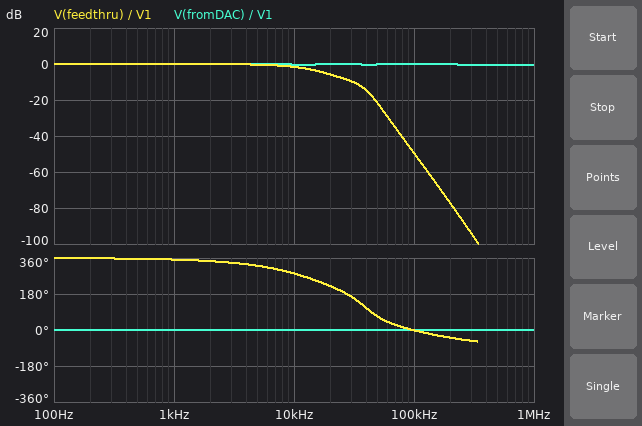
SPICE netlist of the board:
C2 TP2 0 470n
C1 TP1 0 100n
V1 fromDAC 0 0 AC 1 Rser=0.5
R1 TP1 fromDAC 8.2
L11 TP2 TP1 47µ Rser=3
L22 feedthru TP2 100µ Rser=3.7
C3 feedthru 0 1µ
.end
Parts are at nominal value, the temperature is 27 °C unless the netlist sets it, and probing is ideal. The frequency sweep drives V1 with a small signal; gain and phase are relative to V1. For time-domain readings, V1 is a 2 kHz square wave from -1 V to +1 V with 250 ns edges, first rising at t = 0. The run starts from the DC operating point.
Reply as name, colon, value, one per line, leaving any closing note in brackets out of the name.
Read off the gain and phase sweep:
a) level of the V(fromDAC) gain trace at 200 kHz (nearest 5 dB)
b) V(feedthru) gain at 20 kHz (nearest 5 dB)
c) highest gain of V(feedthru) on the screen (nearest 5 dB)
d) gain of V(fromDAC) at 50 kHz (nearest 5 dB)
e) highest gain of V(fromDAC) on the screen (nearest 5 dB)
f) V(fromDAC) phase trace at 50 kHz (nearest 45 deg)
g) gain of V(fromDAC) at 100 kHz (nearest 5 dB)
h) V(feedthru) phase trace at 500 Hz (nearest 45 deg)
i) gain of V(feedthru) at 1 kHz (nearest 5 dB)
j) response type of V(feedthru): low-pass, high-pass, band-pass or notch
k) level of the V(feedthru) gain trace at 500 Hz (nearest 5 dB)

level of the V(fromDAC) gain trace at 200 kHz: 0 dB
V(feedthru) gain at 20 kHz: -5 dB
highest gain of V(feedthru) on the screen: 0 dB
gain of V(fromDAC) at 50 kHz: 0 dB
highest gain of V(fromDAC) on the screen: 0 dB
V(fromDAC) phase trace at 50 kHz: 0 deg
gain of V(fromDAC) at 100 kHz: 0 dB
V(feedthru) phase trace at 500 Hz: 360 deg
gain of V(feedthru) at 1 kHz: 0 dB
response type of V(feedthru): low-pass, high-pass, band-pass or notch: low-pass
level of the V(feedthru) gain trace at 500 Hz: 0 dB
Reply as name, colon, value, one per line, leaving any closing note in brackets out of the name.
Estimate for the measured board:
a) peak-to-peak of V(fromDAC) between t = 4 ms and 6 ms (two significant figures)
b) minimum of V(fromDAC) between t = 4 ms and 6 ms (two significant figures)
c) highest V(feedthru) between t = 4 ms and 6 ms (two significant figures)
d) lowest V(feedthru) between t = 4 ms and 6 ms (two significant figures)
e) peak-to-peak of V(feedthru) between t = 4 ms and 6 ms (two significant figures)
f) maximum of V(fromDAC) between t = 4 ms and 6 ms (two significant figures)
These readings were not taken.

peak-to-peak of V(fromDAC) between t = 4 ms and 6 ms: 2.0 V
minimum of V(fromDAC) between t = 4 ms and 6 ms: -1.0 V
highest V(feedthru) between t = 4 ms and 6 ms: 1.0 V
lowest V(feedthru) between t = 4 ms and 6 ms: -1.0 V
peak-to-peak of V(feedthru) between t = 4 ms and 6 ms: 2.0 V
maximum of V(fromDAC) between t = 4 ms and 6 ms: 1.0 V
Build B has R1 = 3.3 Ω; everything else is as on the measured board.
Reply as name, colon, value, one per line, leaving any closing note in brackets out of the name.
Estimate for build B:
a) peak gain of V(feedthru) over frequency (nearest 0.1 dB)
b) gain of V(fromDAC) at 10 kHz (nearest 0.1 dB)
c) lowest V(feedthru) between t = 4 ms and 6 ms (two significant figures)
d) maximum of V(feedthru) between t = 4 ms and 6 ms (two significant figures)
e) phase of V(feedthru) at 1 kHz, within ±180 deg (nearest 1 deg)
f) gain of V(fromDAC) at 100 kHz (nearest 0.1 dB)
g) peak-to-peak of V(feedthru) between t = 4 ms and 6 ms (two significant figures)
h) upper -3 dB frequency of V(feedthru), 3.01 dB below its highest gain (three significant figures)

peak gain of V(feedthru) over frequency: 1.6 dB
gain of V(fromDAC) at 10 kHz: -0.4 dB
lowest V(feedthru) between t = 4 ms and 6 ms: -1.4 V
maximum of V(feedthru) between t = 4 ms and 6 ms: 1.4 V
phase of V(feedthru) at 1 kHz, within ±180 deg: -5 deg
gain of V(fromDAC) at 100 kHz: 0 dB
peak-to-peak of V(feedthru) between t = 4 ms and 6 ms: 2.7 V
upper -3 dB frequency of V(feedthru), 3.01 dB below its highest gain: 16.4 kHz
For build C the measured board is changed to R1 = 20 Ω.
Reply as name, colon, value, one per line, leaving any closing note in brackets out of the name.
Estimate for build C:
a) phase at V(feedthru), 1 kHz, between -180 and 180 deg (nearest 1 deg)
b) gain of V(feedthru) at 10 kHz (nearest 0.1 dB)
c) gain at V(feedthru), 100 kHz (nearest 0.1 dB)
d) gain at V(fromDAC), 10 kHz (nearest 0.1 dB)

phase at V(feedthru), 1 kHz, between -180 and 180 deg: -14 deg
gain of V(feedthru) at 10 kHz: -6.7 dB
gain at V(feedthru), 100 kHz: -50.6 dB
gain at V(fromDAC), 10 kHz: -0.2 dB
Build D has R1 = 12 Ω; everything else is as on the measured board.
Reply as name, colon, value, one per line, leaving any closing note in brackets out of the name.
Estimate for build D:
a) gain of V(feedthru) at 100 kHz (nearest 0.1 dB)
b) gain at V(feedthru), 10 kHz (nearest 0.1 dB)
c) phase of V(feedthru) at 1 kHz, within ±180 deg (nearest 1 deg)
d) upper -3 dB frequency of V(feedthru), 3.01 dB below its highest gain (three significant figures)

gain of V(feedthru) at 100 kHz: -49.8 dB
gain at V(feedthru), 10 kHz: -3.6 dB
phase of V(feedthru) at 1 kHz, within ±180 deg: -10 deg
upper -3 dB frequency of V(feedthru), 3.01 dB below its highest gain: 8.77 kHz
